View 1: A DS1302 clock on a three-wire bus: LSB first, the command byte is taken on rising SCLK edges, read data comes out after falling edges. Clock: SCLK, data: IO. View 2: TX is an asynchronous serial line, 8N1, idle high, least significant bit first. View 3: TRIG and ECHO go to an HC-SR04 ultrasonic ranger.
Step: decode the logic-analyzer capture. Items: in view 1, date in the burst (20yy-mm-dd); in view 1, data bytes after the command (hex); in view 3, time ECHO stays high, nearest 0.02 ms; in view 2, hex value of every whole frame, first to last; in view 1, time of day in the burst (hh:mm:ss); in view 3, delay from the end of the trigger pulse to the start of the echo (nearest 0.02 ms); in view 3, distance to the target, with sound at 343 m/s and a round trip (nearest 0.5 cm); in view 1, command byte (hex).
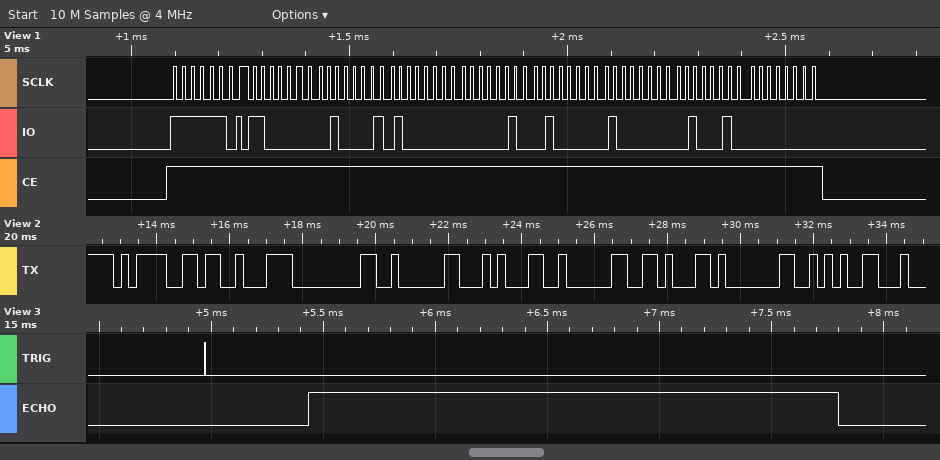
2022-02-20
03 42 01 20 02 01 22 00
2.36 ms
3D 13 00 02 14 02 16 01 2A
01:42:03
0.46 ms
40.5 cm
0xBF
